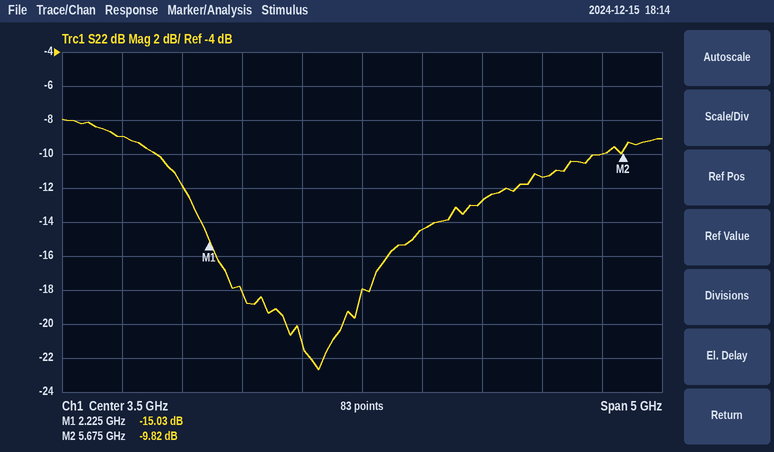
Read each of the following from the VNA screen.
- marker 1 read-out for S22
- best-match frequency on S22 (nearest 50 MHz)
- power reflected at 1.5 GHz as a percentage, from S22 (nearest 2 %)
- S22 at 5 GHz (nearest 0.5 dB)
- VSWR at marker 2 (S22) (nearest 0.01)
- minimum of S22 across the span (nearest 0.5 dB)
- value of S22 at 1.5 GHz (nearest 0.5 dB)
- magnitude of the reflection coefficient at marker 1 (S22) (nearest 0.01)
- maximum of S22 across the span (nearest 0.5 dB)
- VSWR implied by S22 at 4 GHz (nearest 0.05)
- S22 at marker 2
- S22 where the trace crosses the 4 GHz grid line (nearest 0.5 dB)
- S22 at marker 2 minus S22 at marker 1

-15.03 dB
3.15 GHz
12 %
-11.5 dB
1.95
-22.5 dB
-9.0 dB
0.18
-8.0 dB
1.45
-9.82 dB
-14.5 dB
5.21 dB
